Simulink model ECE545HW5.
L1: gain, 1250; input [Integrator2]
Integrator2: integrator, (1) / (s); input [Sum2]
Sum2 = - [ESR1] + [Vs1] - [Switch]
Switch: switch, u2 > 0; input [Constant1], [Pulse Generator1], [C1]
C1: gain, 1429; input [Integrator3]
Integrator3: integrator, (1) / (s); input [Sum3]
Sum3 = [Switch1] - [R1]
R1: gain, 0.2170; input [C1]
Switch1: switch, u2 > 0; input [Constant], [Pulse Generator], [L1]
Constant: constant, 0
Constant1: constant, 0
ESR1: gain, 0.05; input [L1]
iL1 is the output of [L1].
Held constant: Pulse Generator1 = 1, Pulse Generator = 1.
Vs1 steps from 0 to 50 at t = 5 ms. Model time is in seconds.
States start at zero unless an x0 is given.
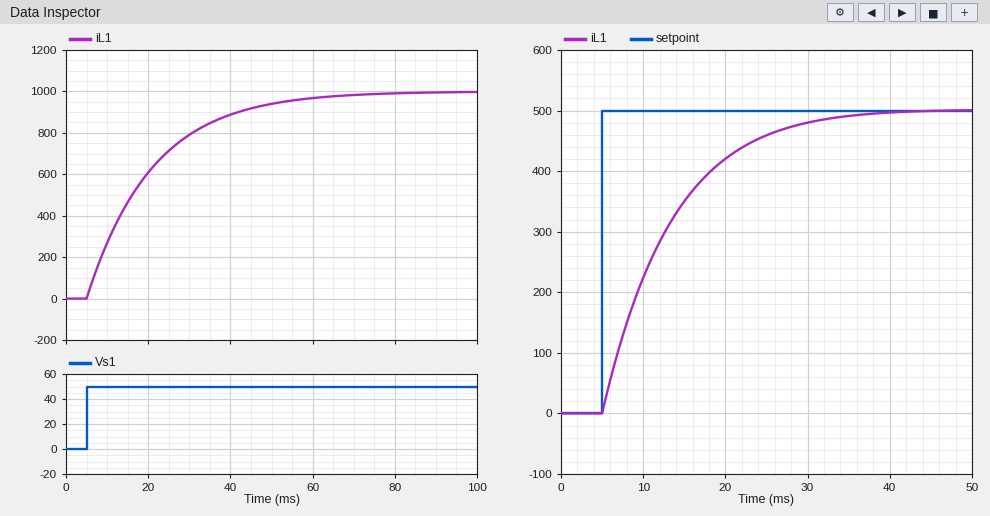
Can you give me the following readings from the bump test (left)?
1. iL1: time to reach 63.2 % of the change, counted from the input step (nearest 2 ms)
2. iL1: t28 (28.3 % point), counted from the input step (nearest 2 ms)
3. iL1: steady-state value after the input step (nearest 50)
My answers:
16 ms
6 ms
1000
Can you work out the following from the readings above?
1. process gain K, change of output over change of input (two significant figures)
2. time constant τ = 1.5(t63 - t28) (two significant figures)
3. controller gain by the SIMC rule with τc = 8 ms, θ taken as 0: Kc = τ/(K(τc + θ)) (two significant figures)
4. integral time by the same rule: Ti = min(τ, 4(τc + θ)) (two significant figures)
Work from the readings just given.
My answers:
20
15 ms
0.094
15 ms
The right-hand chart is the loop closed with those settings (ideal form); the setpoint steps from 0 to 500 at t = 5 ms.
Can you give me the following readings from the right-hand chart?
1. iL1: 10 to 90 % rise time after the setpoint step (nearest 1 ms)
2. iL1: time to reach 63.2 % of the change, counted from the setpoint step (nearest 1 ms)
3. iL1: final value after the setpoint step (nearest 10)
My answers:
18 ms
8 ms
500
